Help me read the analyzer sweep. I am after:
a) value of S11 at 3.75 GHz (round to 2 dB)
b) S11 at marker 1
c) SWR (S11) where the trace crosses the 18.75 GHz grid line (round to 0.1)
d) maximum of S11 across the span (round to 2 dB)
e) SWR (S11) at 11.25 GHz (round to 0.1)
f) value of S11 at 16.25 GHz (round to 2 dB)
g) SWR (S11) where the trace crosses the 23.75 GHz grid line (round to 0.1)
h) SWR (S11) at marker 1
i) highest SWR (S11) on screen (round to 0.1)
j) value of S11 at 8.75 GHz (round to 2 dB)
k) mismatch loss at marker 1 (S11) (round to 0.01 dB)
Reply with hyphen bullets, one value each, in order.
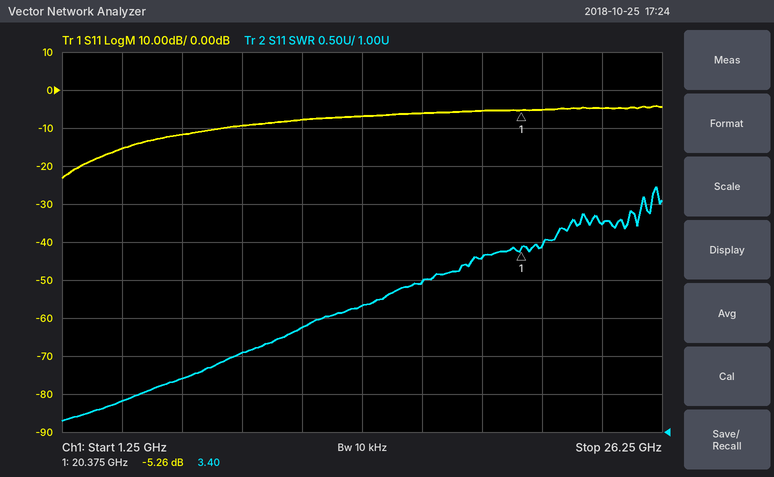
- -16 dB
- -5.26 dB
- 3.3
- -4 dB
- 2.4
- -6 dB
- 3.7
- 3.40
- 4.2
- -10 dB
- 1.54 dB
